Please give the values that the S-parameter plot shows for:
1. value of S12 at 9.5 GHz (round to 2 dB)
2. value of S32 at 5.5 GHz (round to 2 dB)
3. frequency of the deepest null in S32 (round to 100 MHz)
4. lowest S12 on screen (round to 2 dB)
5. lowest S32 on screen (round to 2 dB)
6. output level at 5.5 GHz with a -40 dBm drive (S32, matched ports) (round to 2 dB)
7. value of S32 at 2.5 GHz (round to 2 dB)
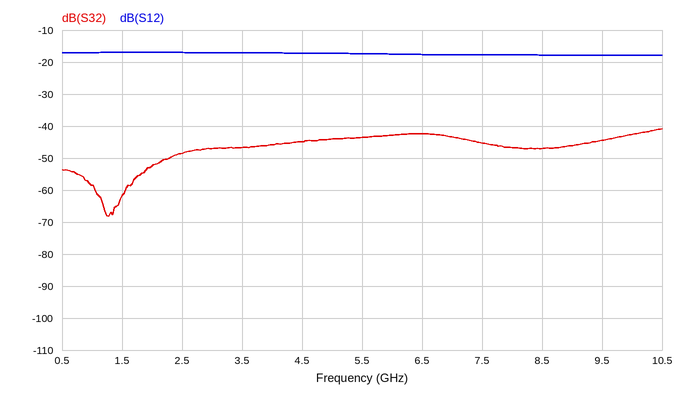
-18 dB
-44 dB
1.3 GHz
-18 dB
-68 dB
-84 dBm
-48 dB
